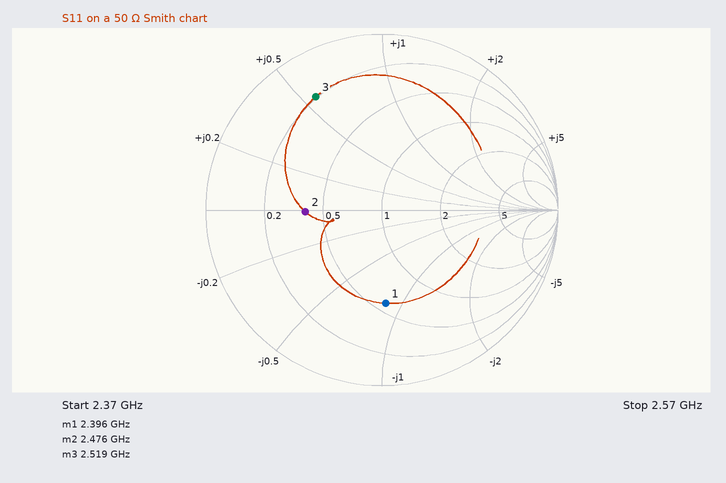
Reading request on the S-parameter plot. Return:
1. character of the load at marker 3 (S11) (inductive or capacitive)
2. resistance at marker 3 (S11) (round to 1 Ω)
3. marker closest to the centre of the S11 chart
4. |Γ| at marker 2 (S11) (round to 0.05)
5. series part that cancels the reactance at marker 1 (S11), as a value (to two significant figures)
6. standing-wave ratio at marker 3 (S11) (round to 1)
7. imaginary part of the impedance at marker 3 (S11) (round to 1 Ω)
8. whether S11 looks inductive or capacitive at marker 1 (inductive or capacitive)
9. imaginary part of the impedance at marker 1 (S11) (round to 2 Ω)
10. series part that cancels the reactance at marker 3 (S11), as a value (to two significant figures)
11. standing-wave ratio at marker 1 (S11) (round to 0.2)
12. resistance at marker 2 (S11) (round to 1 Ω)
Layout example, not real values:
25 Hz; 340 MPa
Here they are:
inductive; 10 Ω; marker 2; 0.45; 2.8 nH; 7; +28 Ω; capacitive; -42 Ω; 2.3 pF; 3.2; 20 Ω
